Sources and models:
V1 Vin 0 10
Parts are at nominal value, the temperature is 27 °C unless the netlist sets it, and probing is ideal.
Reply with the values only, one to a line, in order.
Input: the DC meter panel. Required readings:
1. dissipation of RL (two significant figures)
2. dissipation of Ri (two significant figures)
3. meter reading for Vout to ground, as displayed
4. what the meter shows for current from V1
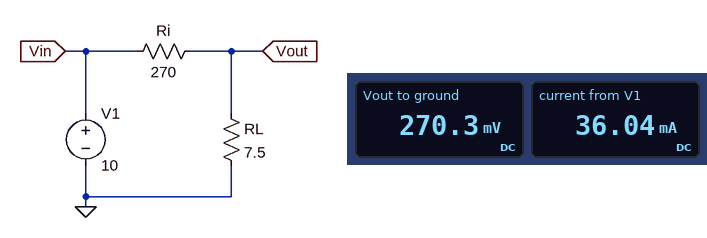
9.7 mW
350 mW
270.3 mV
36.04 mA
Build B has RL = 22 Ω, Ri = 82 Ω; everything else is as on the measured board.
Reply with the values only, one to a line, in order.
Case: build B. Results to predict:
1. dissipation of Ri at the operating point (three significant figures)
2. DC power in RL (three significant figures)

758 mW
203 mW
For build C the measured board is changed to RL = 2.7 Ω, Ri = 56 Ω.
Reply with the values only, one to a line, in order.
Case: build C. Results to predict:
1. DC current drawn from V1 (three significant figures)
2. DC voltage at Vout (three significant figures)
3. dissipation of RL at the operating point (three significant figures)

170 mA
460 mV
78.4 mW
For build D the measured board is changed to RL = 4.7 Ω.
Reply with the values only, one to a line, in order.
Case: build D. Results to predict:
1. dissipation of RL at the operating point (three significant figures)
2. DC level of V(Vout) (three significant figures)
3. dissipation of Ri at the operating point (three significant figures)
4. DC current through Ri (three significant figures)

6.23 mW
171 mV
358 mW
36.4 mA
